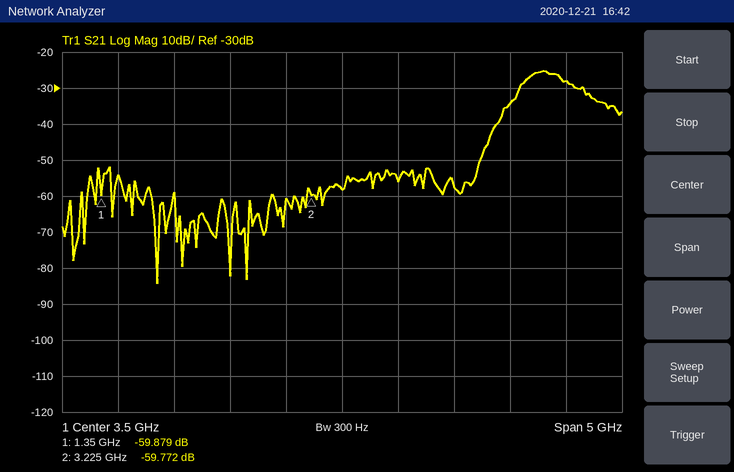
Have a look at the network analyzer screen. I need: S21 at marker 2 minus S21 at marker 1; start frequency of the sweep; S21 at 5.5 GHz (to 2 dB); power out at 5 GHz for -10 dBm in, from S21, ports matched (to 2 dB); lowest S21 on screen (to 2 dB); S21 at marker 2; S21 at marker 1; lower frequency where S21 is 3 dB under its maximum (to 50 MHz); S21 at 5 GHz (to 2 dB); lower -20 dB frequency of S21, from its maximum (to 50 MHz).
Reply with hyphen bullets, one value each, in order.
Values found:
- 0.107 dB
- 1 GHz
- -28 dB
- -44 dBm
- -84 dB
- -59.772 dB
- -59.879 dB
- 5.15 GHz
- -34 dB
- 4.80 GHz
